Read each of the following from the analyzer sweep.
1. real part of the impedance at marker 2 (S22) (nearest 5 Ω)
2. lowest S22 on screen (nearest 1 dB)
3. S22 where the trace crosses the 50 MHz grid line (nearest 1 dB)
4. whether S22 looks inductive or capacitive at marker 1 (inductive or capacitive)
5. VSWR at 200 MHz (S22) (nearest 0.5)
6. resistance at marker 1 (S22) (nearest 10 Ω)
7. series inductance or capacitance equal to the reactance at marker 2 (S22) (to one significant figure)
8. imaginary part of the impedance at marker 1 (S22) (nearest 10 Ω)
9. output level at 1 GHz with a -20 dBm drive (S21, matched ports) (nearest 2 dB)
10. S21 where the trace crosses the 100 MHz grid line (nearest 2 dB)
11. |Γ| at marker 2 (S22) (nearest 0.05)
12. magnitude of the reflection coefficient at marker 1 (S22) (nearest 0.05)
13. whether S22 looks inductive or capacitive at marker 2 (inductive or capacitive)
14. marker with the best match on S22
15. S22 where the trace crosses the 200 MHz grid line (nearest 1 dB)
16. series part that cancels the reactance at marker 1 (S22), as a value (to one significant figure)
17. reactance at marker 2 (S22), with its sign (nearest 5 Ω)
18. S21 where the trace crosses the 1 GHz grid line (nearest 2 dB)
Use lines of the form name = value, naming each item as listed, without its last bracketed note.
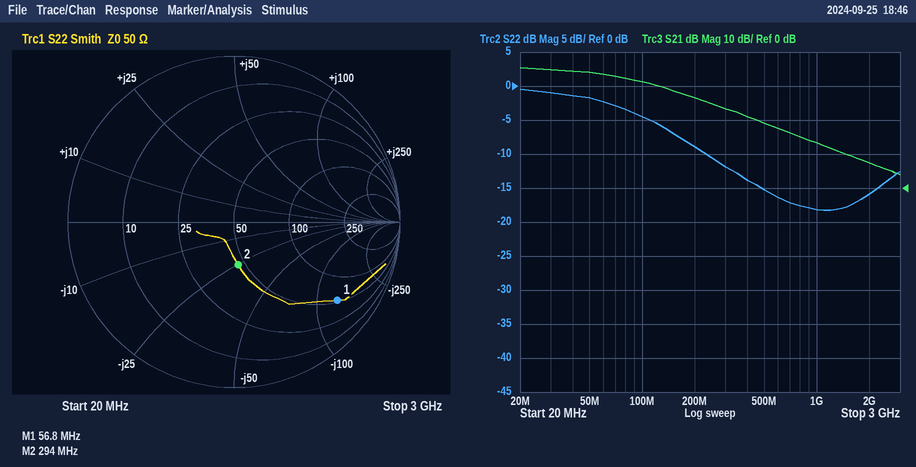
real part of the impedance at marker 2 (S22) = 45 Ω
lowest S22 on screen = -18 dB
S22 where the trace crosses the 50 MHz grid line = -2 dB
whether S22 looks inductive or capacitive at marker 1 = capacitive
VSWR at 200 MHz (S22) = 2.0
resistance at marker 1 (S22) = 50 Ω
series inductance or capacitance equal to the reactance at marker 2 (S22) = 20 pF
imaginary part of the impedance at marker 1 (S22) = -130 Ω
output level at 1 GHz with a -20 dBm drive (S21, matched ports) = -6 dBm
S21 where the trace crosses the 100 MHz grid line = 32 dB
|Γ| at marker 2 (S22) = 0.25
magnitude of the reflection coefficient at marker 1 (S22) = 0.80
whether S22 looks inductive or capacitive at marker 2 = capacitive
marker with the best match on S22 = marker 2
S22 where the trace crosses the 200 MHz grid line = -9 dB
series part that cancels the reactance at marker 1 (S22), as a value = 400 nH
reactance at marker 2 (S22), with its sign = -25 Ω
S21 where the trace crosses the 1 GHz grid line = 14 dB
